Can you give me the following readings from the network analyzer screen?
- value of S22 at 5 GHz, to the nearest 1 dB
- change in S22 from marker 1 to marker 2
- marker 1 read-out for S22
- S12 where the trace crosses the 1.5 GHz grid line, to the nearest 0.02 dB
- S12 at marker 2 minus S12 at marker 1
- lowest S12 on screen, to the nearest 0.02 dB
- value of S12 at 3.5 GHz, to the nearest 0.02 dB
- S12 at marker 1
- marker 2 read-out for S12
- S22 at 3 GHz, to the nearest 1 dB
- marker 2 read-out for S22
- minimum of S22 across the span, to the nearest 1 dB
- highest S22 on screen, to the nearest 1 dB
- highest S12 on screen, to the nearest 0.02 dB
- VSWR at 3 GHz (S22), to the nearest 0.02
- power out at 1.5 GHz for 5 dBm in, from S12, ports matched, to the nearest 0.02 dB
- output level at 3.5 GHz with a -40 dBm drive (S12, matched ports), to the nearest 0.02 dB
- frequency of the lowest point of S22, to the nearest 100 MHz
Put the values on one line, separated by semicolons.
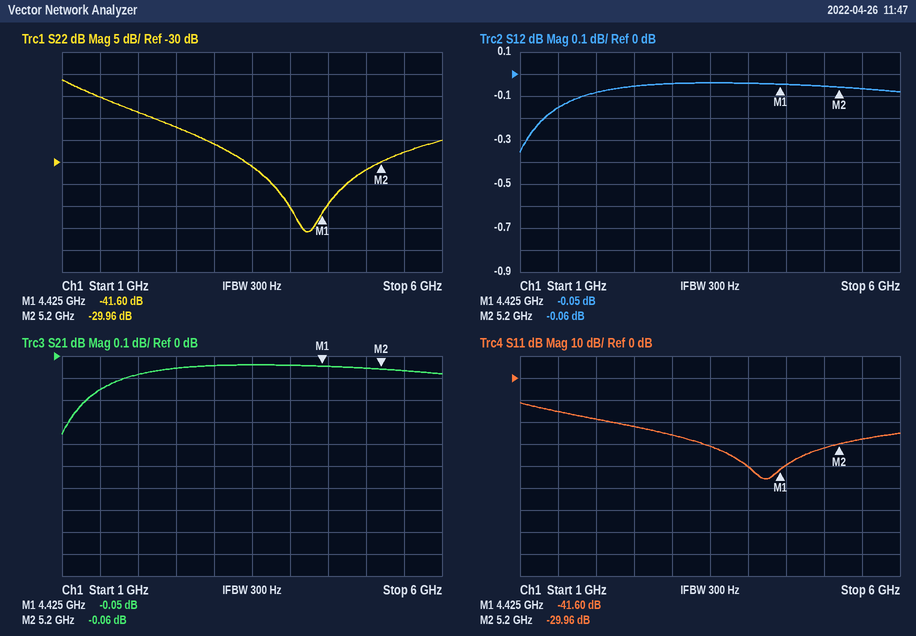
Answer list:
-32 dB; 11.64 dB; -41.60 dB; -0.16 dB; -0.01 dB; -0.36 dB; -0.04 dB; -0.05 dB; -0.06 dB; -26 dB; -29.96 dB; -46 dB; -11 dB; -0.04 dB; 1.10; 4.84 dBm; -40.04 dBm; 4.2 GHz
